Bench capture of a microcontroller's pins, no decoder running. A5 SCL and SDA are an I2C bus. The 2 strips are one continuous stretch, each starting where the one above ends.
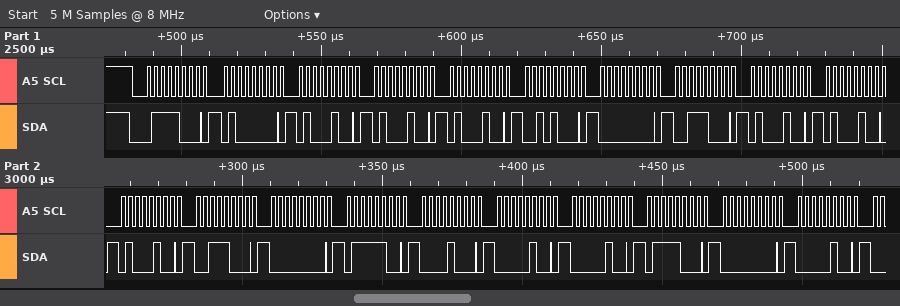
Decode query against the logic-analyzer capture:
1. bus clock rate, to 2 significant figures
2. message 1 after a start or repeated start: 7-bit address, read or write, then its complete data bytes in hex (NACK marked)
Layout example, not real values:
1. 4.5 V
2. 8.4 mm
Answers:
1. 400 kHz
2. 0x3C write: 40 44 44 44 28 00 38 44 44 44 38 00 7C 08 04 04 78 00 04
